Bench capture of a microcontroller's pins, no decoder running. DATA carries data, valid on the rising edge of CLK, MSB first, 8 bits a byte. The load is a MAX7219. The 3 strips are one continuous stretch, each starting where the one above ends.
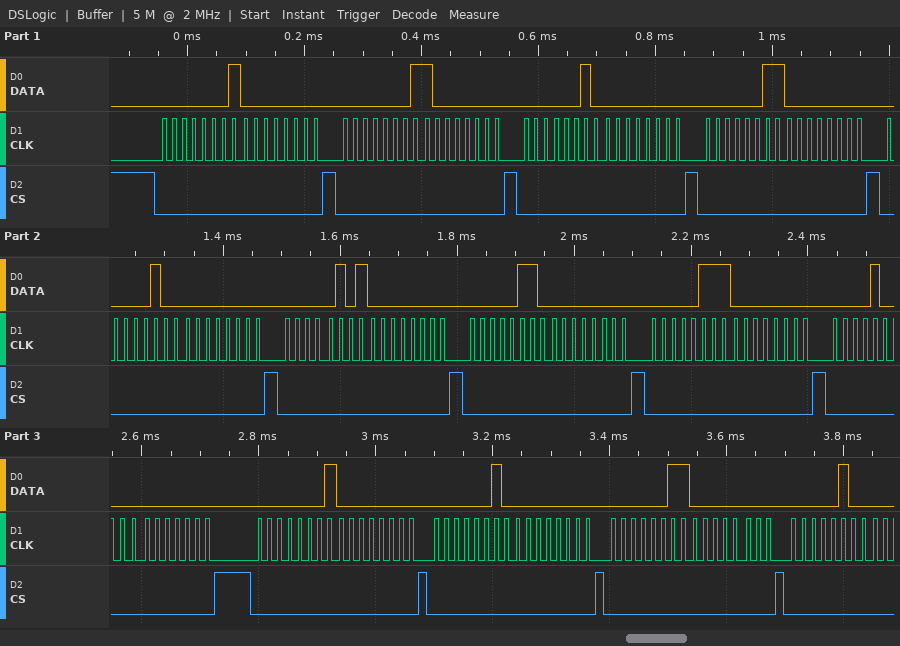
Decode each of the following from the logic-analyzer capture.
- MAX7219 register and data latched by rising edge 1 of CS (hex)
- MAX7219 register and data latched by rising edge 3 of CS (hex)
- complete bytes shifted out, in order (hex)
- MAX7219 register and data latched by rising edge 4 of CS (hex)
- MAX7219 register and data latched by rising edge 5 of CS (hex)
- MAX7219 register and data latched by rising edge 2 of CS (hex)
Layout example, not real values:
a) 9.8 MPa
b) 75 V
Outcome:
a) register 0x1, data 0x00
b) register 0x2, data 0x00
c) 01 00 01 80 02 00 03 00 04 00 05 00 06 00 07 00 08 00 01 00 02 00 03 00 04
d) register 0x3, data 0x00
e) register 0x4, data 0x00
f) register 0x1, data 0x80
